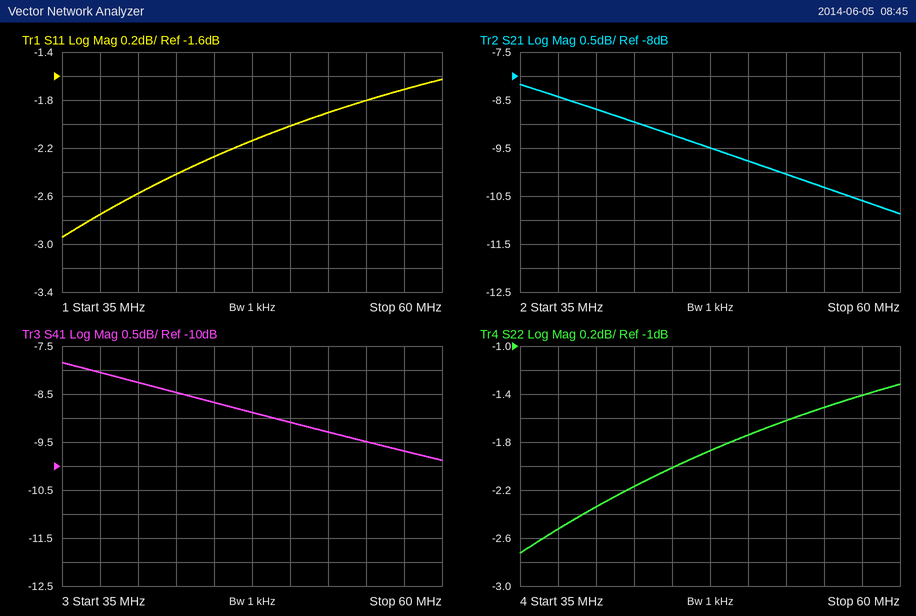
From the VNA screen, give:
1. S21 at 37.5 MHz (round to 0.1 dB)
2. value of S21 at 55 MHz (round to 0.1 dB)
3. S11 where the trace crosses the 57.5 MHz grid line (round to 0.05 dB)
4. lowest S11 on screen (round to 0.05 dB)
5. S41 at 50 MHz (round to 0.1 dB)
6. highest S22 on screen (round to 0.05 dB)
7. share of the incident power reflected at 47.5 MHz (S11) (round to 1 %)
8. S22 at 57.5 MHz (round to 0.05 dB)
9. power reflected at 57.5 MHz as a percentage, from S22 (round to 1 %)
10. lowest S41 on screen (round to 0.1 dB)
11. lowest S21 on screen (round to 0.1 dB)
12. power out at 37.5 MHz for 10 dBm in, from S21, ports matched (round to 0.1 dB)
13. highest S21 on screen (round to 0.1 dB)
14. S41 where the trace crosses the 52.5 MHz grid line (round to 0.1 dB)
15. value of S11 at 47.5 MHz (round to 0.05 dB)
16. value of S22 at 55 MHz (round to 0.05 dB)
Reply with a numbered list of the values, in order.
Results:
1. -8.4 dB
2. -10.3 dB
3. -1.70 dB
4. -2.95 dB
5. -9.1 dB
6. -1.30 dB
7. 61 %
8. -1.40 dB
9. 72 %
10. -9.9 dB
11. -10.9 dB
12. 1.6 dBm
13. -8.2 dB
14. -9.3 dB
15. -2.15 dB
16. -1.50 dB
